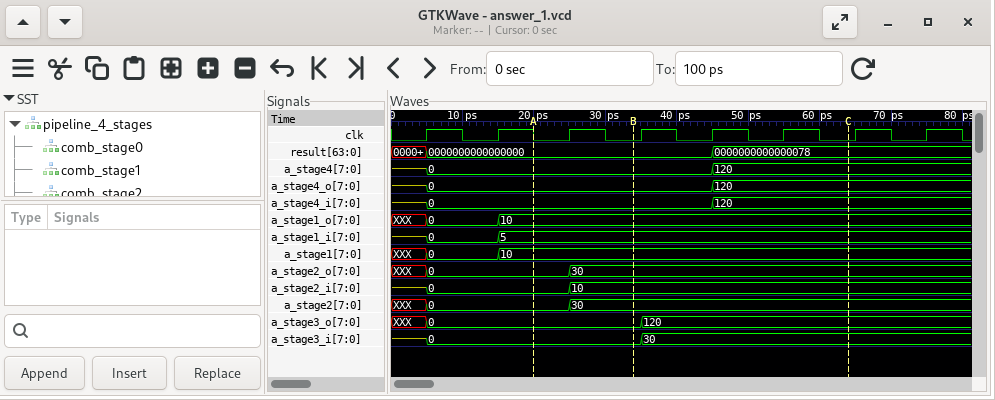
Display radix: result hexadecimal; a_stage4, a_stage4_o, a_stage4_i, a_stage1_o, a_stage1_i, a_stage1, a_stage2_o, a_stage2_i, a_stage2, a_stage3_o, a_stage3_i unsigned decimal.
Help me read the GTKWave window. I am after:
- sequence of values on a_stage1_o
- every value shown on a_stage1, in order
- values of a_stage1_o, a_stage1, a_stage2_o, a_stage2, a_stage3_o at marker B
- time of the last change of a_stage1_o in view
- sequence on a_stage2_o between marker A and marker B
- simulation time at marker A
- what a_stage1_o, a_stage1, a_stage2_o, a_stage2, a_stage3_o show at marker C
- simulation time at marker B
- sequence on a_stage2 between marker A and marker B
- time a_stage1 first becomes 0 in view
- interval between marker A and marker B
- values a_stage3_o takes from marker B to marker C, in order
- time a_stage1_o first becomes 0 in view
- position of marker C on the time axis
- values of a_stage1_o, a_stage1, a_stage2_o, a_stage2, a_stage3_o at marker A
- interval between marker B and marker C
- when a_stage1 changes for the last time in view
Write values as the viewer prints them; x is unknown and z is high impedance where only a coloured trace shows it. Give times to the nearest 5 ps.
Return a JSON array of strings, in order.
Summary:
["XXX, 0, 10", "XXX, 0, 10", "a_stage1_o=10, a_stage1=10, a_stage2_o=30, a_stage2=30, a_stage3_o=0", "15 ps", "0, 30", "20 ps", "a_stage1_o=10, a_stage1=10, a_stage2_o=30, a_stage2=30, a_stage3_o=120", "35 ps", "0, 30", "5 ps", "15 ps", "0, 120", "5 ps", "65 ps", "a_stage1_o=10, a_stage1=10, a_stage2_o=0, a_stage2=0, a_stage3_o=0", "30 ps", "15 ps"]
